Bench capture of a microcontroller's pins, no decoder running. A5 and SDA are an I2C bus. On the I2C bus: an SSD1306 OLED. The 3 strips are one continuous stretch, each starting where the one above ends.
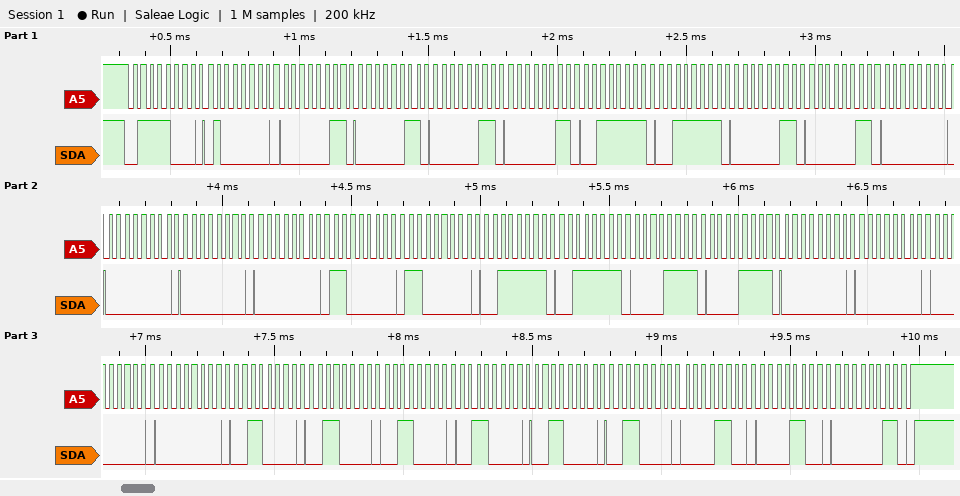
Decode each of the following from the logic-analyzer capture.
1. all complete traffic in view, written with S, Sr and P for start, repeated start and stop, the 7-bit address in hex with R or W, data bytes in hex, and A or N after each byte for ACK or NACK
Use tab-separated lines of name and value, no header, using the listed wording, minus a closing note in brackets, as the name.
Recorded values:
all complete traffic in view, written with S, Sr and P for start, repeated start and stop, the 7-bit address in hex with R or W, data bytes in hex, and A or N after each byte for ACK or NACK	S 3CW A 40 A 03 A 03 A 03 A 03 A 3F A 3F A 03 A 03 A 00 A 00 A 00 A 00 A C0 A C0 A 3F A 3F A 0F A 0F A 00 A 00 A 00 A 00 A 30 A 30 A 30 A 30 A 30 A 30 A 0C A 0C A 03 A P
